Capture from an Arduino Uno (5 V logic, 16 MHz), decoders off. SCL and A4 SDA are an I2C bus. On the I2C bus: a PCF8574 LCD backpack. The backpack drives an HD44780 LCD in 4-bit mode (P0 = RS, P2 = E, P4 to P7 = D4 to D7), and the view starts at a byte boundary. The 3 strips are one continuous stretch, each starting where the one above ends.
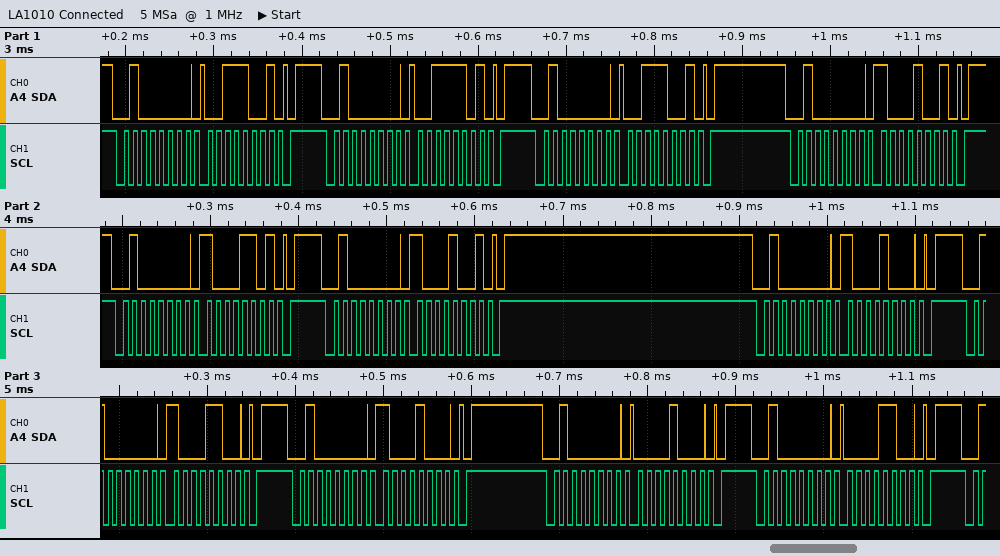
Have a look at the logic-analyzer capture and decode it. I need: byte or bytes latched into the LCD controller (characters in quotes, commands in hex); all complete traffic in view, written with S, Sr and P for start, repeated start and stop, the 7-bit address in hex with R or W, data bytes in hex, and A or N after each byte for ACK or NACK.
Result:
'8'
S 20W A 39 A P S 20W A 3D A P S 20W A 39 A P S 20W A 89 A P S 20W A 8D A P S 20W A 89 A P S 20W A 88 A P S 20W A 8C A P S 20W A 88 A P S 20W A 08 A P S 20W A 0C A P
